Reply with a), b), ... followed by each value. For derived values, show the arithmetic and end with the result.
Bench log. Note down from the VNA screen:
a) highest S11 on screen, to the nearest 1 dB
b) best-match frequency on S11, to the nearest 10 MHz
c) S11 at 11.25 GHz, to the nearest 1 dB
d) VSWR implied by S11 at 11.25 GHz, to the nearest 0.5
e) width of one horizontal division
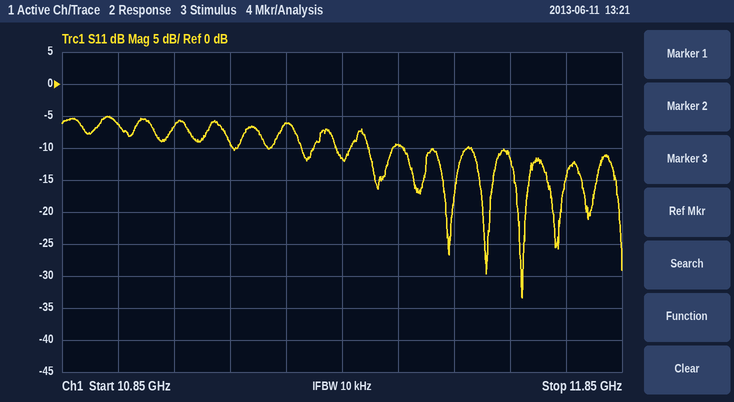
a) -5 dB
b) 11.67 GHz
c) -6 dB
d) |Γ| = 10^(-6/20) = 0.5012; VSWR = (1 + 0.5012)/(1 − 0.5012) ≈ 3.0
e) 100 MHz
